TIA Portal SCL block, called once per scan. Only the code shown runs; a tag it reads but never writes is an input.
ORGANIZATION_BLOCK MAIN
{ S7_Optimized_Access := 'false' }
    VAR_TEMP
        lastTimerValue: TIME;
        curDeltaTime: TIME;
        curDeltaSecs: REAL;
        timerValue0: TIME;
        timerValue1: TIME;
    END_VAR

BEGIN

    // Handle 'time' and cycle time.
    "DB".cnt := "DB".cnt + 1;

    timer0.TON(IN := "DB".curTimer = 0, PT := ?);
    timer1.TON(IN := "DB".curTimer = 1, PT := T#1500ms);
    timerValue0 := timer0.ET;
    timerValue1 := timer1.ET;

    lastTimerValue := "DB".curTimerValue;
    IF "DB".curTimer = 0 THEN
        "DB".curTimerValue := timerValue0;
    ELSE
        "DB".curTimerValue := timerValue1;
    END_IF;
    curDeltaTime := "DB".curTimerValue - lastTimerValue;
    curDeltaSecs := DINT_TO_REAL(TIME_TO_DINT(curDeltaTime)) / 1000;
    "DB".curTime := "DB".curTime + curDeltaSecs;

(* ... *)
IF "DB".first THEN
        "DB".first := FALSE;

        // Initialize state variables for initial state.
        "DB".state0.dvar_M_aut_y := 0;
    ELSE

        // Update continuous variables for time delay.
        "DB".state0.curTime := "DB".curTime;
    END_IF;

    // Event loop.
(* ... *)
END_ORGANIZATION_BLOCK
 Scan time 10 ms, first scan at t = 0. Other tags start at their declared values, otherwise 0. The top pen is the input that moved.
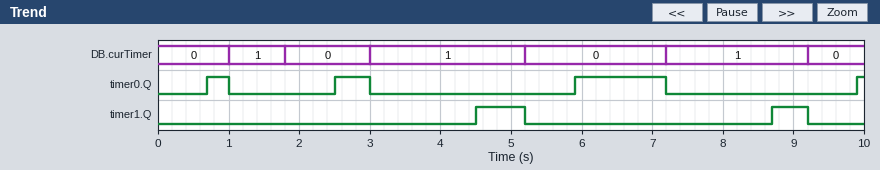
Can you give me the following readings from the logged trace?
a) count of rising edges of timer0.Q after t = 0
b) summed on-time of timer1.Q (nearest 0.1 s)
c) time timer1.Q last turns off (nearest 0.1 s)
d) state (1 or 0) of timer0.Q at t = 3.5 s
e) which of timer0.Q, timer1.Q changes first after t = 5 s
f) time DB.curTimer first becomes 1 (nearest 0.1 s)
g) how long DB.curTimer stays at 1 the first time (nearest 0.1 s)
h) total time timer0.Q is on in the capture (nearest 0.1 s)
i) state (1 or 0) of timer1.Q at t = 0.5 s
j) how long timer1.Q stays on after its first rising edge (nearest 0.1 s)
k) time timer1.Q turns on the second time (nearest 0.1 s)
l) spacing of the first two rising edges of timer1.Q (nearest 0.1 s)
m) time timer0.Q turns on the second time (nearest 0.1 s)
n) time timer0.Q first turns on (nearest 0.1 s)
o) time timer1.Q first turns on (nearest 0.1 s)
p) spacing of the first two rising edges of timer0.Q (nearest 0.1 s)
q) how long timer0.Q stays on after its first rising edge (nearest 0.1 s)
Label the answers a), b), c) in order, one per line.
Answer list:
a) 4
b) 1.2 s
c) 9.2 s
d) 0
e) timer1.Q
f) 1.0 s
g) 0.8 s
h) 2.2 s
i) 0
j) 0.7 s
k) 8.7 s
l) 4.2 s
m) 2.5 s
n) 0.7 s
o) 4.5 s
p) 1.8 s
q) 0.3 s
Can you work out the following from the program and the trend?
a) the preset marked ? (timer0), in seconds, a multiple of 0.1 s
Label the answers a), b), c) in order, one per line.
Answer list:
a) 0.7 s
